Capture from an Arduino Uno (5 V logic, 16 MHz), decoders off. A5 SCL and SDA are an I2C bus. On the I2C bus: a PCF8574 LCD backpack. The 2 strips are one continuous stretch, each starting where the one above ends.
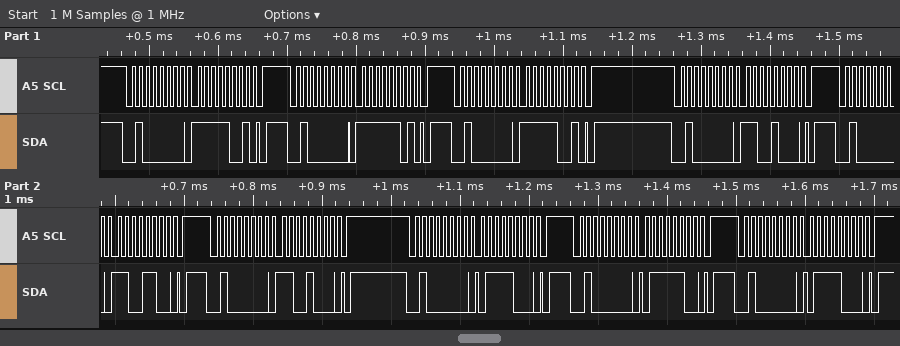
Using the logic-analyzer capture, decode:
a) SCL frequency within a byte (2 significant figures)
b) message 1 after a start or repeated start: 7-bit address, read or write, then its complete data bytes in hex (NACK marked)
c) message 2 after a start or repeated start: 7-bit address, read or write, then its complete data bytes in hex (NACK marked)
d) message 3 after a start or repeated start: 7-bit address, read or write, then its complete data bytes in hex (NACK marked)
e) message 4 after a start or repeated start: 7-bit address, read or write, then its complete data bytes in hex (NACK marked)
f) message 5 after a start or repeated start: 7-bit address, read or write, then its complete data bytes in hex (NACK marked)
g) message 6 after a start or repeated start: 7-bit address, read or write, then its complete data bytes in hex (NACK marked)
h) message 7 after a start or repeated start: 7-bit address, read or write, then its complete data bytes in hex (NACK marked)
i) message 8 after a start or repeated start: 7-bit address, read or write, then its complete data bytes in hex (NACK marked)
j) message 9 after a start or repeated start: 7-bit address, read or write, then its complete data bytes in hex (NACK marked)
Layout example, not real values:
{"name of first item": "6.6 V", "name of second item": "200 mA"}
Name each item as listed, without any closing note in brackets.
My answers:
{"SCL frequency within a byte": "100 kHz", "message 1 after a start or repeated start: 7-bit address, read or write, then its complete data bytes in hex": "0x20 write: F9", "message 2 after a start or repeated start: 7-bit address, read or write, then its complete data bytes in hex": "0x20 write: FD", "message 3 after a start or repeated start: 7-bit address, read or write, then its complete data bytes in hex": "0x20 write: F9", "message 4 after a start or repeated start: 7-bit address, read or write, then its complete data bytes in hex": "0x20 write: C8", "message 5 after a start or repeated start: 7-bit address, read or write, then its complete data bytes in hex": "0x20 write: CC", "message 6 after a start or repeated start: 7-bit address, read or write, then its complete data bytes in hex": "0x20 write: C8", "message 7 after a start or repeated start: 7-bit address, read or write, then its complete data bytes in hex": "0x20 write: 78", "message 8 after a start or repeated start: 7-bit address, read or write, then its complete data bytes in hex": "0x20 write: 7C", "message 9 after a start or repeated start: 7-bit address, read or write, then its complete data bytes in hex": "0x20 write: 78"}
